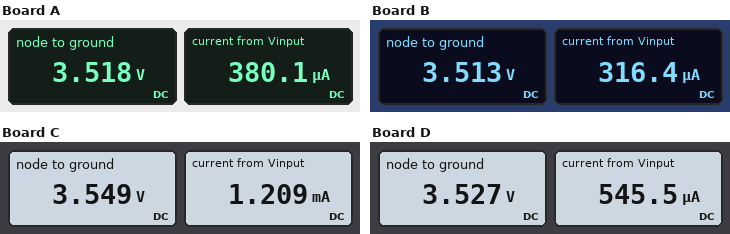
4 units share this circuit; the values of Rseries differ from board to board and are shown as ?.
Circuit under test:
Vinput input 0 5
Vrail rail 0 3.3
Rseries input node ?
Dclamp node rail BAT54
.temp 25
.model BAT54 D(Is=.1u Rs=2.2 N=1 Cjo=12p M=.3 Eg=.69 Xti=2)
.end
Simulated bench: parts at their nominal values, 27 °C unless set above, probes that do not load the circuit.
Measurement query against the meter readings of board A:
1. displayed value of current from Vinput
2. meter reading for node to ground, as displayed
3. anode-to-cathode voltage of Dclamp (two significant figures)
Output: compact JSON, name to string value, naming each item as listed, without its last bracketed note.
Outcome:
{"displayed value of current from Vinput": "380.1 µA", "meter reading for node to ground, as displayed": "3.518 V", "anode-to-cathode voltage of Dclamp": "220 mV"}
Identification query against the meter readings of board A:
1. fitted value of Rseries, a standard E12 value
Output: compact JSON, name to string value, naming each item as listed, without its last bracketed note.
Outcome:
{"fitted value of Rseries, a standard E12 value": "3.9 kΩ"}
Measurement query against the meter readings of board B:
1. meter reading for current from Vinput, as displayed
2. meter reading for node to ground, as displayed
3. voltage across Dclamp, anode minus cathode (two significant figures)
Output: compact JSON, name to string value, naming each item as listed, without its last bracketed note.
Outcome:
{"meter reading for current from Vinput, as displayed": "316.4 µA", "meter reading for node to ground, as displayed": "3.513 V", "voltage across Dclamp, anode minus cathode": "210 mV"}
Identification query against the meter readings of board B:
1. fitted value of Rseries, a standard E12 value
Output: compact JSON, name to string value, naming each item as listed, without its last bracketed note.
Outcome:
{"fitted value of Rseries, a standard E12 value": "4.7 kΩ"}
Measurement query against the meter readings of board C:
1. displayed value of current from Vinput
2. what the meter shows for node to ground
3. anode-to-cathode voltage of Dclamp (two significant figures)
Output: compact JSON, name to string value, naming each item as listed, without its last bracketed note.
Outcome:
{"displayed value of current from Vinput": "1.209 mA", "what the meter shows for node to ground": "3.549 V", "anode-to-cathode voltage of Dclamp": "250 mV"}
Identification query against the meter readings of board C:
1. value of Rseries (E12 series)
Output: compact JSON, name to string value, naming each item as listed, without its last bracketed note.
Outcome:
{"value of Rseries": "1.2 kΩ"}
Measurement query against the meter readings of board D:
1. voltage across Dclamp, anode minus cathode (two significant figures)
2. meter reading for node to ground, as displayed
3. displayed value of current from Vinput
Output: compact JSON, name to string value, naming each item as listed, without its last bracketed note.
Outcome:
{"voltage across Dclamp, anode minus cathode": "230 mV", "meter reading for node to ground, as displayed": "3.527 V", "displayed value of current from Vinput": "545.5 µA"}
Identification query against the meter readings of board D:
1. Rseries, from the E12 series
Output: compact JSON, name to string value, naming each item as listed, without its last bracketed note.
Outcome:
{"Rseries, from the E12 series": "2.7 kΩ"}
